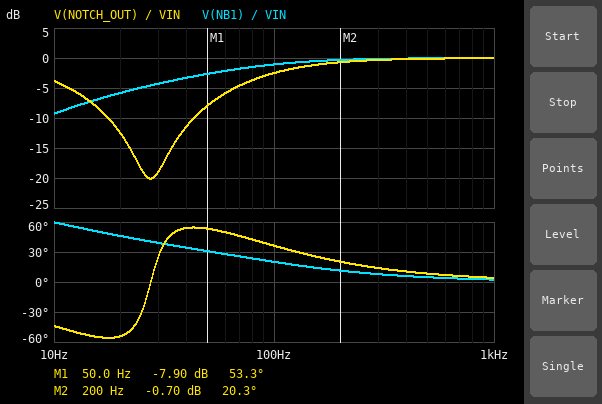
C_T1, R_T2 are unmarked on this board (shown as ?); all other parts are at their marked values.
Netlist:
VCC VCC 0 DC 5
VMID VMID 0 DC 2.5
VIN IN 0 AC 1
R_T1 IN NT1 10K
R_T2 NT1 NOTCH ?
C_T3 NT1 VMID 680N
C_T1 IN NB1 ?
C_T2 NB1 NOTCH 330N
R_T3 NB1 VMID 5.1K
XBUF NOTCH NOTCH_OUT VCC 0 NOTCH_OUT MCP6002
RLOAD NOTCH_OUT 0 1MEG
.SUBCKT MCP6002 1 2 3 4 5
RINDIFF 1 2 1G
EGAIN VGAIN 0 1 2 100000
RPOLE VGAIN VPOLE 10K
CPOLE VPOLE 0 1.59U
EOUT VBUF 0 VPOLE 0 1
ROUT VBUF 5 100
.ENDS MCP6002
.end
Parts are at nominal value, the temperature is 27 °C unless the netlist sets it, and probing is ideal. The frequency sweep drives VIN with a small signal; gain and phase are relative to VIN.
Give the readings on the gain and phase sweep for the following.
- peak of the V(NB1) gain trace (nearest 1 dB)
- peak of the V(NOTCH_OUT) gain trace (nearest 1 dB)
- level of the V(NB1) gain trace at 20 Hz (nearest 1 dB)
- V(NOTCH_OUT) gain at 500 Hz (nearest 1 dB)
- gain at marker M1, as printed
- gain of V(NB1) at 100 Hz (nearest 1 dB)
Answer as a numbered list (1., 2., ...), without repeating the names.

1. 0 dB
2. 0 dB
3. -6 dB
4. 0 dB
5. -7.90 dB
6. -1 dB
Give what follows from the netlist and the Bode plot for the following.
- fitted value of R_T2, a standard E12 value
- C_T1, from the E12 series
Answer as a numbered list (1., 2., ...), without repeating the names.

1. 15 kΩ
2. 1 µF
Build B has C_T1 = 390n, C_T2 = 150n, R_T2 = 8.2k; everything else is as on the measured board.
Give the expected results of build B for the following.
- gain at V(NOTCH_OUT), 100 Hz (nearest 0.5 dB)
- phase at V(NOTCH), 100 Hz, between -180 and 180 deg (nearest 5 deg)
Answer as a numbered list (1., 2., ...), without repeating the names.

1. -13.5 dB
2. 80 deg
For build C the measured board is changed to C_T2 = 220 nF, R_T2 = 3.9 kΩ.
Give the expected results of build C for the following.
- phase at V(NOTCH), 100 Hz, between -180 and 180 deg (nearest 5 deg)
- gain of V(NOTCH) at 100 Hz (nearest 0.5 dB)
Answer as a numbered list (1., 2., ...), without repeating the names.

1. 40 deg
2. -12.0 dB
